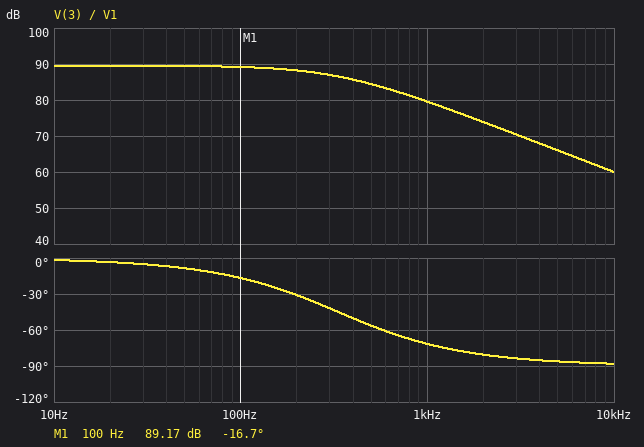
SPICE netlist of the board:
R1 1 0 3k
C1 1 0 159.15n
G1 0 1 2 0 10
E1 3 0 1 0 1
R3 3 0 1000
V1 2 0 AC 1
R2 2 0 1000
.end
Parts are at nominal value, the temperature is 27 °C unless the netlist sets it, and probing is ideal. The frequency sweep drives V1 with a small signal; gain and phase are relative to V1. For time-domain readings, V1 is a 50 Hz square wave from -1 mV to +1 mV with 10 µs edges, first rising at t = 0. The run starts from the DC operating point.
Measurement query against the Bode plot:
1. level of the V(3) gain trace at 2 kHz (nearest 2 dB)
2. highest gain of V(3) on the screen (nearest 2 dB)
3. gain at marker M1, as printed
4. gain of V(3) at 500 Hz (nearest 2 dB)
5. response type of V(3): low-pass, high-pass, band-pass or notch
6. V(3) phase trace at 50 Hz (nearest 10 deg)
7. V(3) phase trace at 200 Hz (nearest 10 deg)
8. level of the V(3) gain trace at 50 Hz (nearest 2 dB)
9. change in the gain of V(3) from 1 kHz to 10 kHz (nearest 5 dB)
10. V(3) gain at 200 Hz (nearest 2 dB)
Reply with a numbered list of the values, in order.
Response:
1. 74 dB
2. 90 dB
3. 89.17 dB
4. 84 dB
5. low-pass
6. -10 deg
7. -30 deg
8. 90 dB
9. -20 dB
10. 88 dB
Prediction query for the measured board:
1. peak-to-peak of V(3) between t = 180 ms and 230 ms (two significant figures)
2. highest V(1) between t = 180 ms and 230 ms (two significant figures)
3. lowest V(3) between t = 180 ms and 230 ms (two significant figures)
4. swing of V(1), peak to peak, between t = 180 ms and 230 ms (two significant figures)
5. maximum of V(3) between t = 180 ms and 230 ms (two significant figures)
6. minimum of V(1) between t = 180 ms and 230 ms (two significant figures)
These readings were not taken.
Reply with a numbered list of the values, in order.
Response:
1. 60 V
2. 30 V
3. -30 V
4. 60 V
5. 30 V
6. -30 V
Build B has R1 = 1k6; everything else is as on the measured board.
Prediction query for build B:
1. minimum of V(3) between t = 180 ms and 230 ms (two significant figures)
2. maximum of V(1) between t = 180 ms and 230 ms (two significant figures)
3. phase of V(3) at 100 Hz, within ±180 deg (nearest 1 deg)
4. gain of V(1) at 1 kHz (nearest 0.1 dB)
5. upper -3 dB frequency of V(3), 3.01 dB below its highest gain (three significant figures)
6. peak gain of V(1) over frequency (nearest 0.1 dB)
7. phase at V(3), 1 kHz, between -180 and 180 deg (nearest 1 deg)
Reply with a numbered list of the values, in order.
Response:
1. -16 V
2. 16 V
3. -9 deg
4. 78.6 dB
5. 625 Hz
6. 84.1 dB
7. -58 deg
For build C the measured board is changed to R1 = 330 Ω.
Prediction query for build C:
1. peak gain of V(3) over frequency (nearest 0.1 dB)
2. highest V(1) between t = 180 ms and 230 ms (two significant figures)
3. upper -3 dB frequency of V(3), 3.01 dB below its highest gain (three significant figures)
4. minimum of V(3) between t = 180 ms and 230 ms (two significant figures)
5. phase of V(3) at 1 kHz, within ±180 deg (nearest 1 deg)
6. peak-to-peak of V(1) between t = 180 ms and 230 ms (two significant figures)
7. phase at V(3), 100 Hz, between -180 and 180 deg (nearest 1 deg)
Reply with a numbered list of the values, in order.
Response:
1. 70.4 dB
2. 3.3 V
3. 3.03 kHz
4. -3.3 V
5. -18 deg
6. 6.6 V
7. -2 deg
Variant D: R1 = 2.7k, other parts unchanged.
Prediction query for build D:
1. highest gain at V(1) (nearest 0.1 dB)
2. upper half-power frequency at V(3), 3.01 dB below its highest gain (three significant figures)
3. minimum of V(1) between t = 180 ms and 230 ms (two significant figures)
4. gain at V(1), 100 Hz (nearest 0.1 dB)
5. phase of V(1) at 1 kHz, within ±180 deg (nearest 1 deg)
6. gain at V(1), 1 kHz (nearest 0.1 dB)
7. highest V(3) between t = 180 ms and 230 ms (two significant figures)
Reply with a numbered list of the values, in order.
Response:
1. 88.6 dB
2. 370 Hz
3. -27 V
4. 88.3 dB
5. -70 deg
6. 79.4 dB
7. 27 V
